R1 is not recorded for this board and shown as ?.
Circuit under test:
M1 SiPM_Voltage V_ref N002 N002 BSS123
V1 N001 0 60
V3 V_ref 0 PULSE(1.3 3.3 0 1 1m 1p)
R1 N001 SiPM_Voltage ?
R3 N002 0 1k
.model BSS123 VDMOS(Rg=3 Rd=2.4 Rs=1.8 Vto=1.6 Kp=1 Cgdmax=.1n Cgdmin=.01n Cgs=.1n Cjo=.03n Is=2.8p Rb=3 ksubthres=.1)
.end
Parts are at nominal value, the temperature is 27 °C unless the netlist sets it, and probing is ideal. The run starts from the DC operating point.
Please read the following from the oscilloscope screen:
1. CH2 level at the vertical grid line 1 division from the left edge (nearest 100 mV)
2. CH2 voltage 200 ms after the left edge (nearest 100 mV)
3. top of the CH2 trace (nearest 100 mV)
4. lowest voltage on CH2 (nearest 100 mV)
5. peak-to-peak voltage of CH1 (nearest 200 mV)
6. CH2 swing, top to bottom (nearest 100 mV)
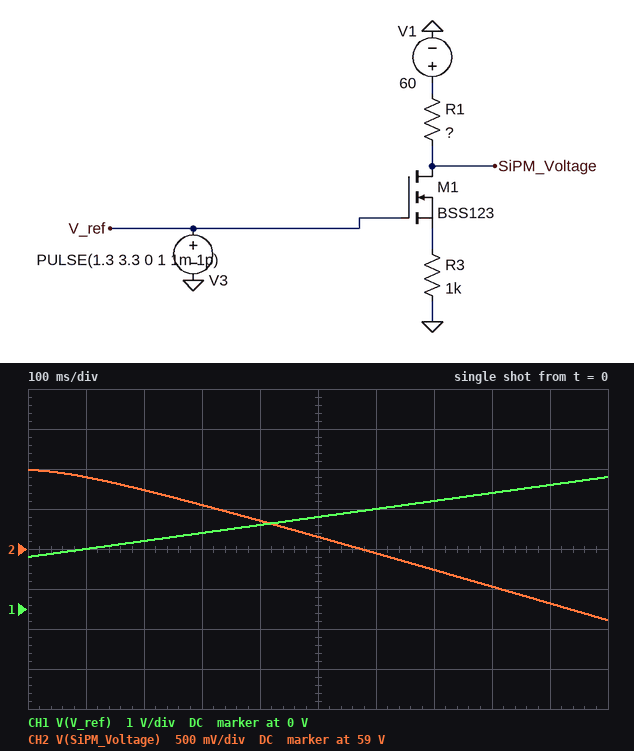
59.9 V
59.7 V
60.0 V
58.1 V
2.0 V
1.9 V
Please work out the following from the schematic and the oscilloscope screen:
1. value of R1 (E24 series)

1.1 kΩ
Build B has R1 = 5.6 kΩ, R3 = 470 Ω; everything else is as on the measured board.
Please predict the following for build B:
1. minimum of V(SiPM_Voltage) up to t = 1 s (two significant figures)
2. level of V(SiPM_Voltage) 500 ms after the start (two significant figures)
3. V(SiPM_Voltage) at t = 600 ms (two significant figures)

40 V
51 V
49 V
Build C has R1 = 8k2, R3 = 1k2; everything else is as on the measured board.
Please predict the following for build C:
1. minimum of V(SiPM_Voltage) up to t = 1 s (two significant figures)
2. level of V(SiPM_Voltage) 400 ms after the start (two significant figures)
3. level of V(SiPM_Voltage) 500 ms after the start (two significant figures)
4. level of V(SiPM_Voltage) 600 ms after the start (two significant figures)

48 V
56 V
55 V
53 V
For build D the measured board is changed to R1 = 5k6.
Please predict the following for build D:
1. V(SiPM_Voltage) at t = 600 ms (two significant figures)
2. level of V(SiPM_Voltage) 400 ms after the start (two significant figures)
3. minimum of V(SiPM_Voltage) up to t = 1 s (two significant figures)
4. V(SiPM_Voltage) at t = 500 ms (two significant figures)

55 V
57 V
50 V
56 V
